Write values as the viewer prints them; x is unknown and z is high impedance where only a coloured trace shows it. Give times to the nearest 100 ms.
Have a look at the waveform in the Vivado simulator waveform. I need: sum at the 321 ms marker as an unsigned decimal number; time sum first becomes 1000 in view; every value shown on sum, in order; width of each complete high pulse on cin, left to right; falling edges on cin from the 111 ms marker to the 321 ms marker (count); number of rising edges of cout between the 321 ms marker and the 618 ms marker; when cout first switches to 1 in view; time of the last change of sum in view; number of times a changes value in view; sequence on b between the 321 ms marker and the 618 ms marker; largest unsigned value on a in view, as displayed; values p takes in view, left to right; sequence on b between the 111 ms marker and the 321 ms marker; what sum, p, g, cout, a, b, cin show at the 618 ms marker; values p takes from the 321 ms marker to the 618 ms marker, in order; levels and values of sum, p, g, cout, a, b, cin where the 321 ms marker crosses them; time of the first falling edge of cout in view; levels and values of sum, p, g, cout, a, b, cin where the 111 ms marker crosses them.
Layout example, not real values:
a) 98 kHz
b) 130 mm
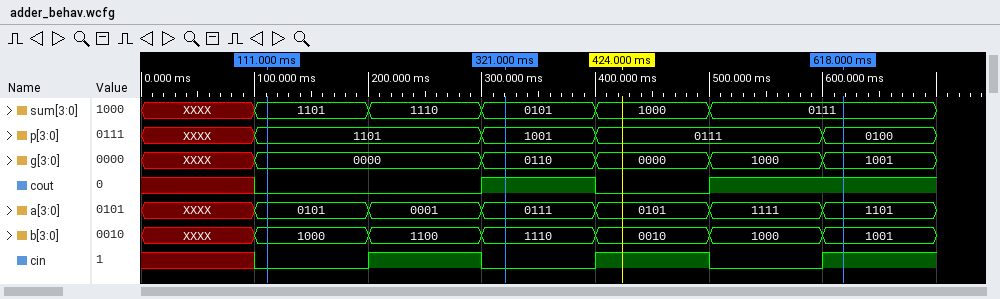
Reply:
a) 5
b) 400 ms
c) XXXX, 1101, 1110, 0101, 1000, 0111
d) 100 ms, 100 ms
e) 1
f) 1
g) 300 ms
h) 500 ms
i) 6
j) 1110, 0010, 1000, 1001
k) 1111
l) XXXX, 1101, 1001, 0111, 0100
m) 1000, 1100, 1110
n) sum=0111, p=0100, g=1001, cout=1, a=1101, b=1001, cin=1
o) 1001, 0111, 0100
p) sum=0101, p=1001, g=0110, cout=1, a=0111, b=1110, cin=0
q) 400 ms
r) sum=1101, p=1101, g=0000, cout=0, a=0101, b=1000, cin=0
